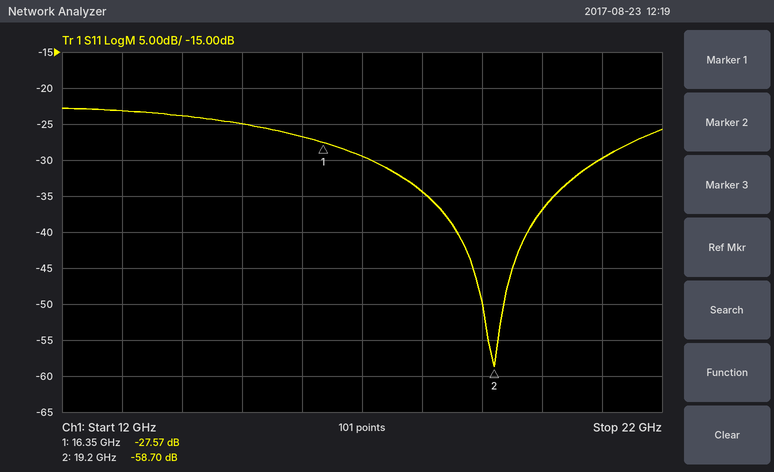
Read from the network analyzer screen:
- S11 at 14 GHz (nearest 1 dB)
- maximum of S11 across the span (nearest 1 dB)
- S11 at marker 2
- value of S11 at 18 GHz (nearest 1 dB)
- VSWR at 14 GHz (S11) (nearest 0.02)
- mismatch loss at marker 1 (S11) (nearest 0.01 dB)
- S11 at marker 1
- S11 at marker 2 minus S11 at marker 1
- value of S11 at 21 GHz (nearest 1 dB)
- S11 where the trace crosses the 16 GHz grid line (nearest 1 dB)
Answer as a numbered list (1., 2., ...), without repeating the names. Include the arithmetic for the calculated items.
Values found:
1. -24 dB
2. -23 dB
3. -58.70 dB
4. -34 dB
5. |Γ| = 10^(-24/20) = 0.0631; VSWR = (1 + 0.0631)/(1 − 0.0631) ≈ 1.13, so 1.14 to the nearest 0.02
6. −10 log10(1 − 10^(-27.57/10)) ≈ 0.01 dB
7. -27.57 dB
8. -58.7 − (-27.57) = -31.13 dB
9. -30 dB
10. -27 dB
